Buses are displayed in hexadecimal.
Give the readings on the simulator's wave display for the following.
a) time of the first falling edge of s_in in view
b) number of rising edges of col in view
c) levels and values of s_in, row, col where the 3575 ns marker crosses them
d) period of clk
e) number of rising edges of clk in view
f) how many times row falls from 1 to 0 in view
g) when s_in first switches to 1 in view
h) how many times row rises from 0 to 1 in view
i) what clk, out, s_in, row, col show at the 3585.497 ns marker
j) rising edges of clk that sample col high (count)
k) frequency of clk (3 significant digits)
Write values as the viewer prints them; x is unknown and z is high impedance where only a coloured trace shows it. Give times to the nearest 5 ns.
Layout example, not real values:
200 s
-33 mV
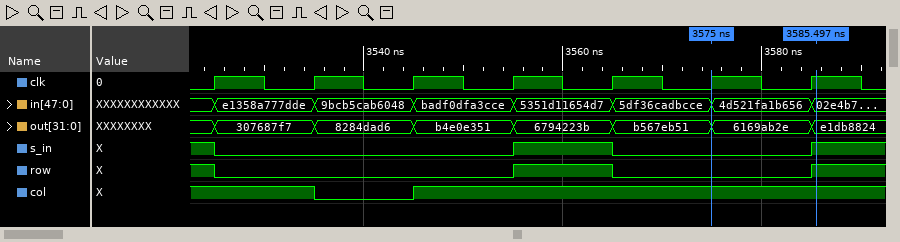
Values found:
3525 ns
1
s_in=0, row=0, col=1
10 ns
7
2
3555 ns
2
clk=1, out=e1db8824, s_in=1, row=1, col=1
6
100 MHz
